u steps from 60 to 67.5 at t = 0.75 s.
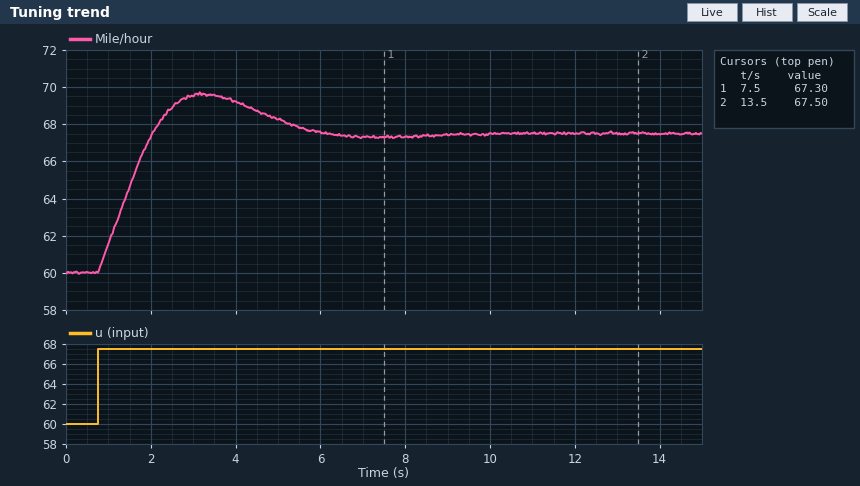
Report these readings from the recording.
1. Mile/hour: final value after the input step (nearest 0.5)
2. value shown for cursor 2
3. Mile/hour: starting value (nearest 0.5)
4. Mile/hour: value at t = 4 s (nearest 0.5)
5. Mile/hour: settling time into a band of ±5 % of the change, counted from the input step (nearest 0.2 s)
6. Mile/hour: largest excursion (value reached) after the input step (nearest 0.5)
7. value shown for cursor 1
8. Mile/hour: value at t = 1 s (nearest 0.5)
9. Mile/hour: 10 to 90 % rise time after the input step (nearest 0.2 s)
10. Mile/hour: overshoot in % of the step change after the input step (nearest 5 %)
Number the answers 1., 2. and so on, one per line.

1. 67.5
2. 67.50
3. 60.0
4. 69.0
5. 4.8 s
6. 69.5
7. 67.30
8. 61.5
9. 1.0 s
10. 30 %
